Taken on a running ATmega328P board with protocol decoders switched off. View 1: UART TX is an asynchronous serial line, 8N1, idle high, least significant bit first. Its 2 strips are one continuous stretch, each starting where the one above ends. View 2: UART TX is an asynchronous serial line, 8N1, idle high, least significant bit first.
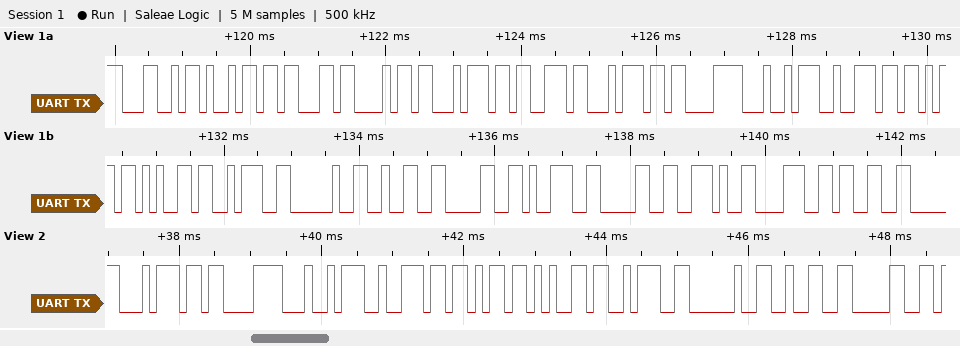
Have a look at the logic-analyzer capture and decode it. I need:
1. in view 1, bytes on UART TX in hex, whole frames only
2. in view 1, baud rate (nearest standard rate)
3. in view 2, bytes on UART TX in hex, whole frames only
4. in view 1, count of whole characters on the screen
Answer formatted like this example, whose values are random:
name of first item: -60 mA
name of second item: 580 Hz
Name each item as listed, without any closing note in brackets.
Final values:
in view 1, bytes on UART TX in hex, whole frames only: 4C 69 63 68 74 73 74 C3 A4 72 6B 65 3A 20 32 30 39 30 2E 38 33
in view 1, baud rate: 9600 baud
in view 2, bytes on UART TX in hex, whole frames only: 74 C3 A4 72 6B 65 3A 20 32 30
in view 1, count of whole characters on the screen: 21
